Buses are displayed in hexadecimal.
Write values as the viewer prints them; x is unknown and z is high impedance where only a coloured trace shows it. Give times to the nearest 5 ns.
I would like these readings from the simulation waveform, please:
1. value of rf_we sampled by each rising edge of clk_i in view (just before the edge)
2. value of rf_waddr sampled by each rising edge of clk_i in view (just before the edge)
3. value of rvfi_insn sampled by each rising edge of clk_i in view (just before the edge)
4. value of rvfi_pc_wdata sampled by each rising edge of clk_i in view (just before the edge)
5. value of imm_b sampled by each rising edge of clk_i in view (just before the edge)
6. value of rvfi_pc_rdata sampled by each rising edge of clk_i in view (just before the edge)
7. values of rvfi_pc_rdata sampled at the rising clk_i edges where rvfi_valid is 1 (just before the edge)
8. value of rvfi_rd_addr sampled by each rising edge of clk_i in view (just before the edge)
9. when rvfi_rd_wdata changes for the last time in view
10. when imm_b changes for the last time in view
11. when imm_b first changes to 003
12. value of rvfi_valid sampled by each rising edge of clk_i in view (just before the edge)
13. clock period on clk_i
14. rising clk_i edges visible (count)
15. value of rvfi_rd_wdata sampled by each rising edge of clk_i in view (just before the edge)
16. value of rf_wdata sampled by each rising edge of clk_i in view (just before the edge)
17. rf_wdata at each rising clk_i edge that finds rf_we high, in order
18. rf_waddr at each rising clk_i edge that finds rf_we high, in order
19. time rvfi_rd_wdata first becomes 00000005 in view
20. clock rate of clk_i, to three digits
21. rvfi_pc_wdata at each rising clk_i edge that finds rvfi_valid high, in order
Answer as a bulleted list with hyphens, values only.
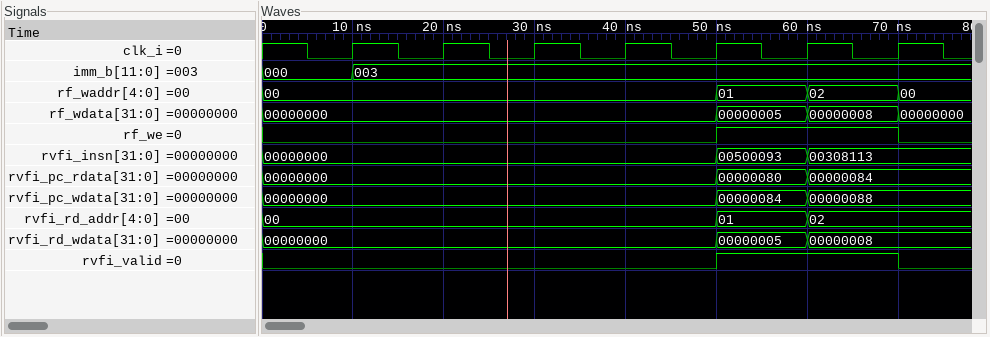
- 0 0 0 0 0 1 1
- 00, 00, 00, 00, 00, 01, 02
- 00000000, 00000000, 00000000, 00000000, 00000000, 00500093, 00308113
- 00000000, 00000000, 00000000, 00000000, 00000000, 00000084, 00000088
- 000, 003, 003, 003, 003, 003, 003
- 00000000, 00000000, 00000000, 00000000, 00000000, 00000080, 00000084
- 00000080, 00000084
- 00, 00, 00, 00, 00, 01, 02
- 60 ns
- 10 ns
- 10 ns
- 0 0 0 0 0 1 1
- 10 ns
- 7
- 00000000, 00000000, 00000000, 00000000, 00000000, 00000005, 00000008
- 00000000, 00000000, 00000000, 00000000, 00000000, 00000005, 00000008
- 00000005, 00000008
- 01, 02
- 50 ns
- 100 MHz
- 00000084, 00000088
